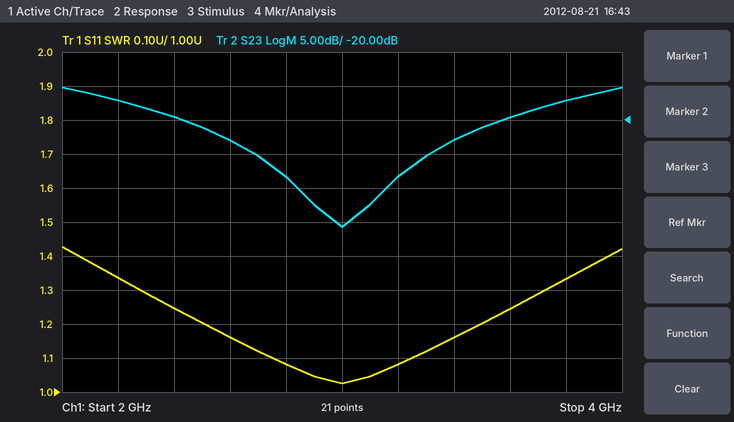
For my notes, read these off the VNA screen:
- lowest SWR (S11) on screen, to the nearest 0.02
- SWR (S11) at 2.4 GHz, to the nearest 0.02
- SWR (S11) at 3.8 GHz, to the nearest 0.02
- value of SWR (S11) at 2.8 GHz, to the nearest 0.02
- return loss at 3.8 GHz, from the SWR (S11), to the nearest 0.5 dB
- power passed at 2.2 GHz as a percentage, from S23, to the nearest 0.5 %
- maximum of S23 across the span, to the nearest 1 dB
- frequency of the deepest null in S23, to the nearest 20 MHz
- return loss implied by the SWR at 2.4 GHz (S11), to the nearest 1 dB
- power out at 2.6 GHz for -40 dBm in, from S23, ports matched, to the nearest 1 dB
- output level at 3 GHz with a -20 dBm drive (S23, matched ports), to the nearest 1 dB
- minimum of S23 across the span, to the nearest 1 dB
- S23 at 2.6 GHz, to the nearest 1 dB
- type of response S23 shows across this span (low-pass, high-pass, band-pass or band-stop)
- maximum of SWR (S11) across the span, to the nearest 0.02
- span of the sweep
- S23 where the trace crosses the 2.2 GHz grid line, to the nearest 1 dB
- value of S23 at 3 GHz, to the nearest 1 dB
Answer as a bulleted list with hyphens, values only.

- 1.02
- 1.24
- 1.34
- 1.08
- 17.0 dB
- 2.0 %
- -15 dB
- 3.00 GHz
- 19 dB
- -63 dBm
- -56 dBm
- -36 dB
- -23 dB
- band-stop
- 1.42
- 2 GHz
- -17 dB
- -36 dB
